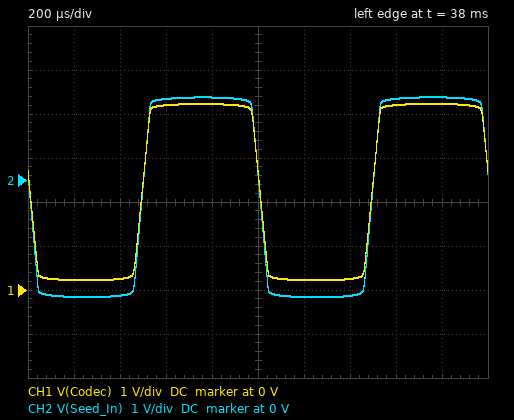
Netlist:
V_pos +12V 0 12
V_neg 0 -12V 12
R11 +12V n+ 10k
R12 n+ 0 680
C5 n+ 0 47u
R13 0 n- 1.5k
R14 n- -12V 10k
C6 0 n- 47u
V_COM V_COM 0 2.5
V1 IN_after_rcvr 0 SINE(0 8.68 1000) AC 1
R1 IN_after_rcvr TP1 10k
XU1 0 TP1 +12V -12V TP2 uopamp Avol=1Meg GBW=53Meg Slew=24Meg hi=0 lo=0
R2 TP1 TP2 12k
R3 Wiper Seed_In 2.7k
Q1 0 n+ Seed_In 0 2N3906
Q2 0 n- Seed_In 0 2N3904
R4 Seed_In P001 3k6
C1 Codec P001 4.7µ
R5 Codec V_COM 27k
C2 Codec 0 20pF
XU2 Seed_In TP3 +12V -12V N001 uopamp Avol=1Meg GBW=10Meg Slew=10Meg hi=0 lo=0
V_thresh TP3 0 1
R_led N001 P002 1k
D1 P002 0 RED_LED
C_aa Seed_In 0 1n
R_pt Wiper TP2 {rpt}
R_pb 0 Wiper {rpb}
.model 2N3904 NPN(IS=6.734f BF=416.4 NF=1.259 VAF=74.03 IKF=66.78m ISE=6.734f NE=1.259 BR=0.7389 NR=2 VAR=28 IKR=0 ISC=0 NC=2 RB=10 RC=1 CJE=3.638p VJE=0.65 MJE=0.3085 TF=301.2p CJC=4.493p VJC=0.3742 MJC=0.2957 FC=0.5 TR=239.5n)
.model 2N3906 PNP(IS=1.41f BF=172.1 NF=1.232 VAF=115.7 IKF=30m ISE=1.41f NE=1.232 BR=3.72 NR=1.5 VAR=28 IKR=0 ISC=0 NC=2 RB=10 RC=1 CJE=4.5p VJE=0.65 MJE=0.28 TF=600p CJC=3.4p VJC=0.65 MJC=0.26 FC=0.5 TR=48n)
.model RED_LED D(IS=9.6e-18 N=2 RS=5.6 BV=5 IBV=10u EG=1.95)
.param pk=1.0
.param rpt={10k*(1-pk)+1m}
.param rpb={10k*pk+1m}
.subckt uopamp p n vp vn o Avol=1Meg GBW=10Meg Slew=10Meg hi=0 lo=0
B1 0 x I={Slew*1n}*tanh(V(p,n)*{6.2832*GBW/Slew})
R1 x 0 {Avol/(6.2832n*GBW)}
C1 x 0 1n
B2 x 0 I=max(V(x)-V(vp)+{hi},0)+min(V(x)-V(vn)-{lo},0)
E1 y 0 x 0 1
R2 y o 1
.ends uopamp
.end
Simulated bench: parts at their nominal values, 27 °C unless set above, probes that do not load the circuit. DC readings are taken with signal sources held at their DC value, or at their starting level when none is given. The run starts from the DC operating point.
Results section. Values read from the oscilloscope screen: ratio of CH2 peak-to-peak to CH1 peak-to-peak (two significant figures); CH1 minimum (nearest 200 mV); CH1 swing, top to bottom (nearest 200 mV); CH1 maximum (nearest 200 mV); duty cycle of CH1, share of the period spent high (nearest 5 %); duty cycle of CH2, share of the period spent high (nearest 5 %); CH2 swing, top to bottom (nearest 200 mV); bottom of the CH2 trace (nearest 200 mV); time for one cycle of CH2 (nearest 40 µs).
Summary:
1.1
200 mV
4.0 V
4.2 V
50 %
50 %
4.6 V
-2.6 V
1.00 ms
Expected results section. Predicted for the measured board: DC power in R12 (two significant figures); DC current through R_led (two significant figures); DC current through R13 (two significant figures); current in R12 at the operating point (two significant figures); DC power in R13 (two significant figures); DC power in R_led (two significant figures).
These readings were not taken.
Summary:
860 µW
6.6 mA
1.0 mA
1.1 mA
1.6 mW
44 mW
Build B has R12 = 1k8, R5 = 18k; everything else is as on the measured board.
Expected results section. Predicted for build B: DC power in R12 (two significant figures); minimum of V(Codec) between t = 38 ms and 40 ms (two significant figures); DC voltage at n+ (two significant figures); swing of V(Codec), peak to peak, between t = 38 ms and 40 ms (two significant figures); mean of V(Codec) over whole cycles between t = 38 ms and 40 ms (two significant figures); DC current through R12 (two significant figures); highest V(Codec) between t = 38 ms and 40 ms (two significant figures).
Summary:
1.9 mW
250 mV
1.8 V
4.7 V
2.6 V
1.0 mA
4.9 V
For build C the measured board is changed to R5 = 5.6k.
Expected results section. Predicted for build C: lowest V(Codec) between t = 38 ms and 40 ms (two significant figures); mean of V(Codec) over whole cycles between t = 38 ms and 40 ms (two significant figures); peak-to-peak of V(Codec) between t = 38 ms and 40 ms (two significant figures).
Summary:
1.0 V
2.4 V
2.7 V
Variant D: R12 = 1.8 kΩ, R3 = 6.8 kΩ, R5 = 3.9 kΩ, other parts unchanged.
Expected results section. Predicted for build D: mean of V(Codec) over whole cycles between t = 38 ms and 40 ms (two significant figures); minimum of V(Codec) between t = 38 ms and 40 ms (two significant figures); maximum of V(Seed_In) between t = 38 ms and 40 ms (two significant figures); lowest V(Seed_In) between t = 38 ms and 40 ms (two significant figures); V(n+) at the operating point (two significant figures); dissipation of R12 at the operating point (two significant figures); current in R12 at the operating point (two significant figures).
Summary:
2.5 V
1.2 V
2.7 V
-2.4 V
1.8 V
1.9 mW
1.0 mA
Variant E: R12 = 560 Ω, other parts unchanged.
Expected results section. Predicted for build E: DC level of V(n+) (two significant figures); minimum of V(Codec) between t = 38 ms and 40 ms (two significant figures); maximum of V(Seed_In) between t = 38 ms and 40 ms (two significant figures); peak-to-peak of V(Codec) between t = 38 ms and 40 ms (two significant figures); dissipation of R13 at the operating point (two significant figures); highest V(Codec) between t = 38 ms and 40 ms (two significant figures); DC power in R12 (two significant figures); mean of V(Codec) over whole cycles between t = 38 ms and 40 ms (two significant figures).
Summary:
640 mV
230 mV
1.7 V
3.9 V
1.6 mW
4.1 V
720 µW
2.2 V
